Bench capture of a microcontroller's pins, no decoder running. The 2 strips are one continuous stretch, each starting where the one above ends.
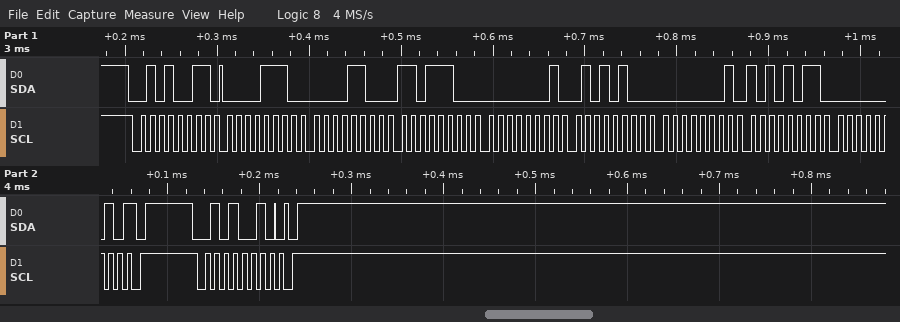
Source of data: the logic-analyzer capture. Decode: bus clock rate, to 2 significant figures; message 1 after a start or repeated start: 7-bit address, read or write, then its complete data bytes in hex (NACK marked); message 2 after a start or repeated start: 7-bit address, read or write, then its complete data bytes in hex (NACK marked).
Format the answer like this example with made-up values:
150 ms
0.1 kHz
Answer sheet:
100 kHz
0x29 read: 0E 0C DC 01 54 01 AB 02 NACK
0x29 write
